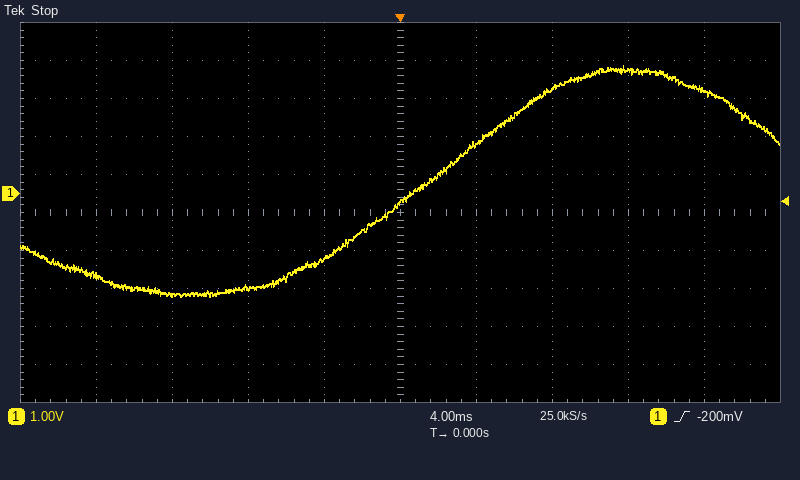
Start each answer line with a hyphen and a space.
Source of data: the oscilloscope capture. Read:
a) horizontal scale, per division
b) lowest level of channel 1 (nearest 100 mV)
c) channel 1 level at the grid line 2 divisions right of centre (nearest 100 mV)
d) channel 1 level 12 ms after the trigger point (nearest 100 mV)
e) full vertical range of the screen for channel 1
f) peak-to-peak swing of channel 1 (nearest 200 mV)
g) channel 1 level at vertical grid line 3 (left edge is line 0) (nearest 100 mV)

- 4 ms
- -2.7 V
- 2.8 V
- 3.2 V
- 10 V
- 6.0 V
- -2.5 V
